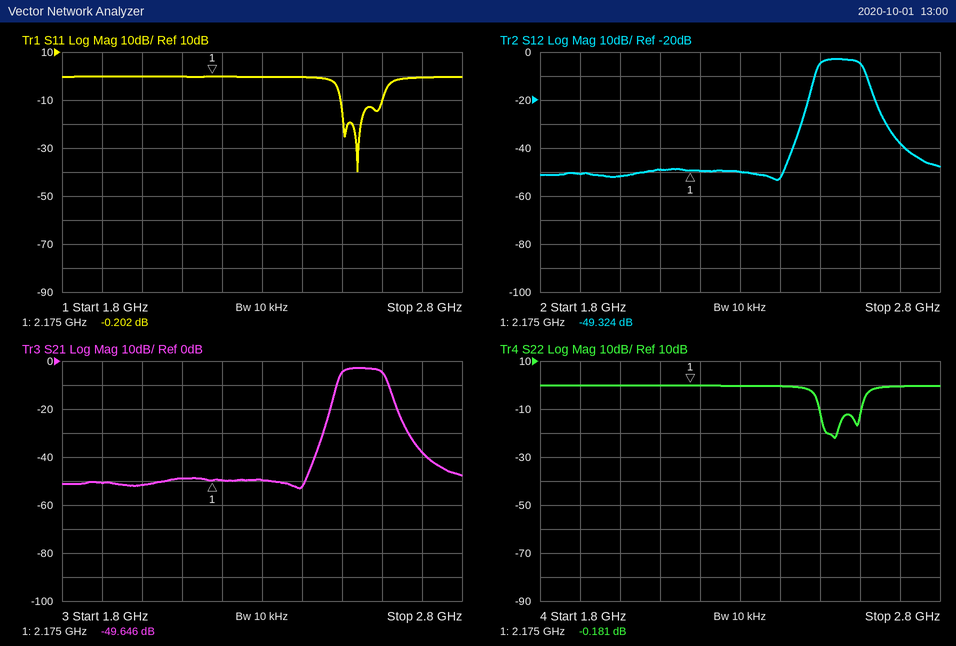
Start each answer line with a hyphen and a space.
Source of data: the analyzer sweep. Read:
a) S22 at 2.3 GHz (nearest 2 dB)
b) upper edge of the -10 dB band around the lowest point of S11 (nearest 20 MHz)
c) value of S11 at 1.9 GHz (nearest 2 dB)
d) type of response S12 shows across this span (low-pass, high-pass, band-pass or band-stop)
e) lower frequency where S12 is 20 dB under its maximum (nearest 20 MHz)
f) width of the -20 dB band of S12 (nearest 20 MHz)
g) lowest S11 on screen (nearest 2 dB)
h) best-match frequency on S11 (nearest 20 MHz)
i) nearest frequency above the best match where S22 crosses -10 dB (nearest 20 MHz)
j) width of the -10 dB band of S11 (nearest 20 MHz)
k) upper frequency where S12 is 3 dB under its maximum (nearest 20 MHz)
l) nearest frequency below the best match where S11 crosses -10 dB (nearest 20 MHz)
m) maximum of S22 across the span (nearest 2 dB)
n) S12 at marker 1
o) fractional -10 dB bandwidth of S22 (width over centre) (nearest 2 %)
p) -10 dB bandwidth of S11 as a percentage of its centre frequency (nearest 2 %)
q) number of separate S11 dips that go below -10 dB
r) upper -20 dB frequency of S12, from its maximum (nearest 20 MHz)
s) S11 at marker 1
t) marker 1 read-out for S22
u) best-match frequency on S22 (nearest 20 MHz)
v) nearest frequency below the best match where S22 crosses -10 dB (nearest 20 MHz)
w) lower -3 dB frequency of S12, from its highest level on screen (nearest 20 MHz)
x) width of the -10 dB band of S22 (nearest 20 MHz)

- 0 dB
- 2.60 GHz
- 0 dB
- band-pass
- 2.46 GHz
- 180 MHz
- -40 dB
- 2.54 GHz
- 2.60 GHz
- 100 MHz
- 2.60 GHz
- 2.50 GHz
- 0 dB
- -49.324 dB
- 4 %
- 4 %
- 2
- 2.64 GHz
- -0.202 dB
- -0.181 dB
- 2.54 GHz
- 2.50 GHz
- 2.50 GHz
- 100 MHz
